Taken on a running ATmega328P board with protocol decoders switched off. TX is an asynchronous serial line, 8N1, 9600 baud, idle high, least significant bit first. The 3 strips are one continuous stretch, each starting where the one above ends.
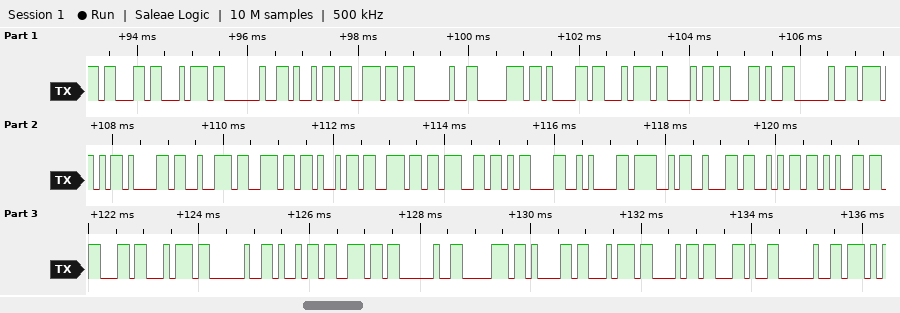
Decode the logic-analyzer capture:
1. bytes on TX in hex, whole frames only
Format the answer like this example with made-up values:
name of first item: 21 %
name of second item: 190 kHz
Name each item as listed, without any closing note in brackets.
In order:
bytes on TX in hex, whole frames only: 63 74 20 69 6E 20 70 61 74 68 2C 20 57 61 72 6E 69 6E 67 0D 0A 4F 62 6A 65 63 74 20 69 6E 20 70 61 74 68 2C 20
